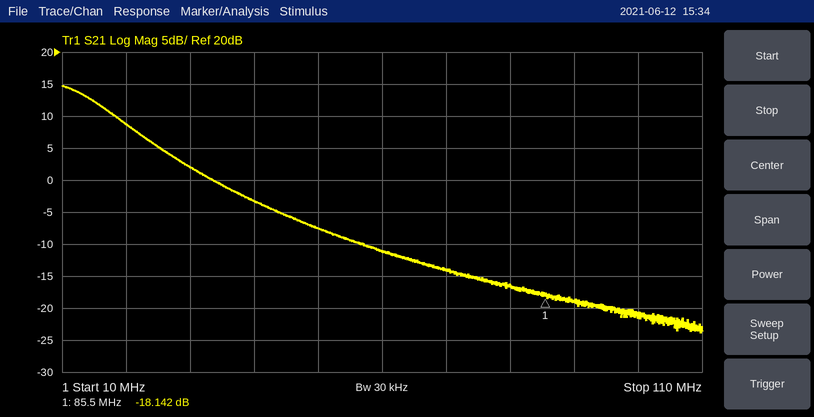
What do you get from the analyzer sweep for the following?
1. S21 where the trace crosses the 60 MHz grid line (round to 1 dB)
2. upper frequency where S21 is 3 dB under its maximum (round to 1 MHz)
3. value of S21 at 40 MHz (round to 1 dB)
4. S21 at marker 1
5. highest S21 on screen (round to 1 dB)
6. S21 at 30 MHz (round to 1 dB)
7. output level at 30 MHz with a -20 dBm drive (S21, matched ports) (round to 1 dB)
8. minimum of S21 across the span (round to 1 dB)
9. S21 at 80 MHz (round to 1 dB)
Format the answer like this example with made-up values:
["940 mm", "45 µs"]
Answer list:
["-11 dB", "16 MHz", "-3 dB", "-18.142 dB", "15 dB", "2 dB", "-18 dBm", "-24 dB", "-16 dB"]
